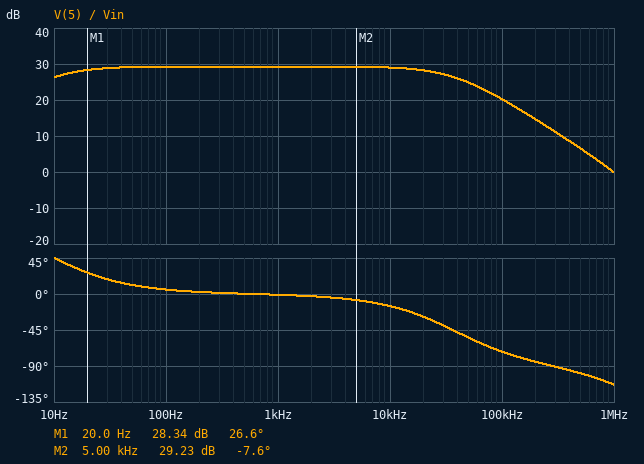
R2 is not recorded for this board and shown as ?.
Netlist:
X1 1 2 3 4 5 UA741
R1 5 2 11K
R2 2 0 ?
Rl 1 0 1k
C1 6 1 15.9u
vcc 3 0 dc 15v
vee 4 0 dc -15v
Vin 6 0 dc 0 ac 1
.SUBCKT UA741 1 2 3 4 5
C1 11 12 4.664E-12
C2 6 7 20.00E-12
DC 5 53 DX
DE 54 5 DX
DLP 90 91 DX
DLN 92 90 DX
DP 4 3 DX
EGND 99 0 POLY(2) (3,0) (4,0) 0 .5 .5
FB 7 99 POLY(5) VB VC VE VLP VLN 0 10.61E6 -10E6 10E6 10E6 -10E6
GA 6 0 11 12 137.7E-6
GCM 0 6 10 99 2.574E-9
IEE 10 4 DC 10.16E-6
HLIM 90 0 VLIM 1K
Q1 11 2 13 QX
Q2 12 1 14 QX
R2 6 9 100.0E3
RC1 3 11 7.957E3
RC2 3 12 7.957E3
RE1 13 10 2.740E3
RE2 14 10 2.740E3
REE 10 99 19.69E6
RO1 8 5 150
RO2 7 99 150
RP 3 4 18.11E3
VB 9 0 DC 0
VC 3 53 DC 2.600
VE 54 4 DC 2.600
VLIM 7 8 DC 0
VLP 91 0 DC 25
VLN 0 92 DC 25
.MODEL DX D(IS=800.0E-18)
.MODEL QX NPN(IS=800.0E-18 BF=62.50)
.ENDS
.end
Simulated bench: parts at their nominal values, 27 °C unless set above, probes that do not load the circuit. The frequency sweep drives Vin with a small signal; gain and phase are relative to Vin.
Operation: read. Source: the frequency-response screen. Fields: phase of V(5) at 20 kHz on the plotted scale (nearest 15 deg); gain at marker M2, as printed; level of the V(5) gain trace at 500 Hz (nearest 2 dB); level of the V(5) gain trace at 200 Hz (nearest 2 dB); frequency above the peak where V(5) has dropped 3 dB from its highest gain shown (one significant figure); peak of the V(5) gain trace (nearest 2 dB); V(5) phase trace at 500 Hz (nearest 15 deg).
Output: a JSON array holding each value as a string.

["-30 deg", "29.23 dB", "30 dB", "30 dB", "40 kHz", "30 dB", "0 deg"]
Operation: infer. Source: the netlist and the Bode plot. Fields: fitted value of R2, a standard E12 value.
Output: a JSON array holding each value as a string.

["390 Ω"]
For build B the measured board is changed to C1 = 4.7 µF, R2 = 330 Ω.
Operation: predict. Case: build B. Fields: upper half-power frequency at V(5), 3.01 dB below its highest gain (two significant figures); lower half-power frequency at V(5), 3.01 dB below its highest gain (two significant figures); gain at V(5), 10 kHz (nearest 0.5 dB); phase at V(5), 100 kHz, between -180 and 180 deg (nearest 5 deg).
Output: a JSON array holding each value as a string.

["32 kHz", "34 Hz", "30.5 dB", "-75 deg"]
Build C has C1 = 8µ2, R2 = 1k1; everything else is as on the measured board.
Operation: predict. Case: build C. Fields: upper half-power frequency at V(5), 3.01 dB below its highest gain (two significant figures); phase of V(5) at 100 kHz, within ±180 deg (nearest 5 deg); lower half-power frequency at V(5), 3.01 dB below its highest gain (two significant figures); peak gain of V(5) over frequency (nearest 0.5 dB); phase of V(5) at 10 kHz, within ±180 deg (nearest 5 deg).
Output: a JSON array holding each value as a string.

["100 kHz", "-45 deg", "19 Hz", "21.0 dB", "-5 deg"]
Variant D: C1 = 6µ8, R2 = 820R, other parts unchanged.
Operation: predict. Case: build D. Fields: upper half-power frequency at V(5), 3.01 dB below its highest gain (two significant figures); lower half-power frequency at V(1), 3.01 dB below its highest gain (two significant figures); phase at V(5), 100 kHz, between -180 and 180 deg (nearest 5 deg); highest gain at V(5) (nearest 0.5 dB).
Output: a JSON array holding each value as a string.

["78 kHz", "23 Hz", "-55 deg", "23.0 dB"]
